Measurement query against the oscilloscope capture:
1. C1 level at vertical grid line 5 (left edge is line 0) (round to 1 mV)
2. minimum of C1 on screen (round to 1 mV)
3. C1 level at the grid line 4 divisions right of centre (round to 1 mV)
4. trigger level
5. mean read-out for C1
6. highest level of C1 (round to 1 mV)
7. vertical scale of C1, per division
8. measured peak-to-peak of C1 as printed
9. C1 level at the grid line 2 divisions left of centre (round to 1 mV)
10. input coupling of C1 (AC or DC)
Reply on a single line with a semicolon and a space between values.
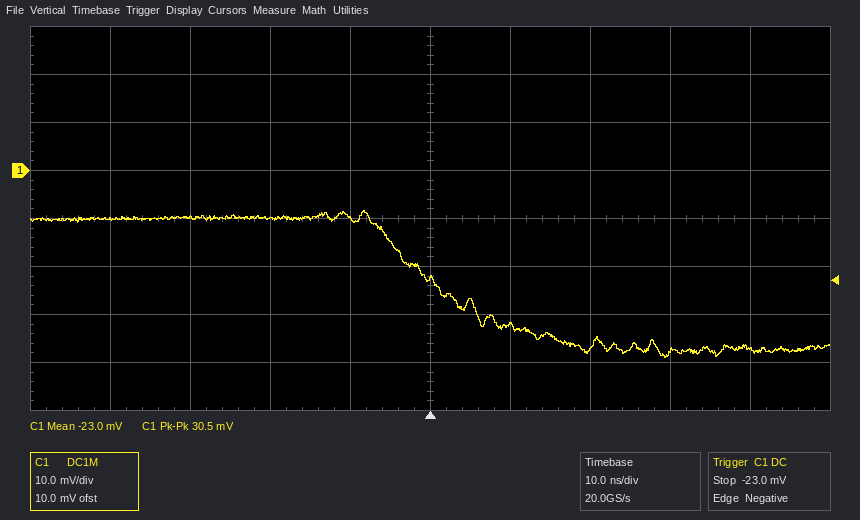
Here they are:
-23 mV; -39 mV; -37 mV; -23.0 mV; -23.0 mV; -8 mV; 10 mV; 30.5 mV; -10 mV; DC
